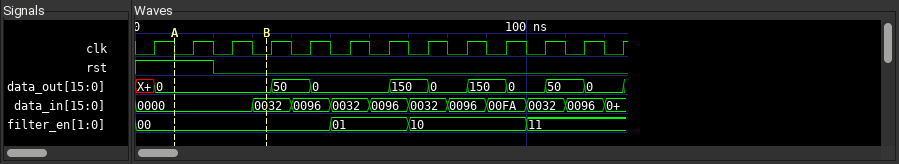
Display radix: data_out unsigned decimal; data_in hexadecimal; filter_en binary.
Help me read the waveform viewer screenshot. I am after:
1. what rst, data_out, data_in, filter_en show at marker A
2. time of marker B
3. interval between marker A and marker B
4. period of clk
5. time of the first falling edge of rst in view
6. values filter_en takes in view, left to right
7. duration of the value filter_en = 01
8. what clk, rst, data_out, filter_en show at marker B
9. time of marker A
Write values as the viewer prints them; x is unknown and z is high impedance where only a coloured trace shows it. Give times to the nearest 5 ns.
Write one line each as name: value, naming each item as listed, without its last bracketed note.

what rst, data_out, data_in, filter_en show at marker A: rst=1, data_out=0, data_in=0000, filter_en=00
time of marker B: 35 ns
interval between marker A and marker B: 25 ns
period of clk: 10 ns
time of the first falling edge of rst in view: 20 ns
values filter_en takes in view, left to right: 00, 01, 10, 11
duration of the value filter_en = 01: 20 ns
what clk, rst, data_out, filter_en show at marker B: clk=0, rst=0, data_out=0, filter_en=00
time of marker A: 10 ns
